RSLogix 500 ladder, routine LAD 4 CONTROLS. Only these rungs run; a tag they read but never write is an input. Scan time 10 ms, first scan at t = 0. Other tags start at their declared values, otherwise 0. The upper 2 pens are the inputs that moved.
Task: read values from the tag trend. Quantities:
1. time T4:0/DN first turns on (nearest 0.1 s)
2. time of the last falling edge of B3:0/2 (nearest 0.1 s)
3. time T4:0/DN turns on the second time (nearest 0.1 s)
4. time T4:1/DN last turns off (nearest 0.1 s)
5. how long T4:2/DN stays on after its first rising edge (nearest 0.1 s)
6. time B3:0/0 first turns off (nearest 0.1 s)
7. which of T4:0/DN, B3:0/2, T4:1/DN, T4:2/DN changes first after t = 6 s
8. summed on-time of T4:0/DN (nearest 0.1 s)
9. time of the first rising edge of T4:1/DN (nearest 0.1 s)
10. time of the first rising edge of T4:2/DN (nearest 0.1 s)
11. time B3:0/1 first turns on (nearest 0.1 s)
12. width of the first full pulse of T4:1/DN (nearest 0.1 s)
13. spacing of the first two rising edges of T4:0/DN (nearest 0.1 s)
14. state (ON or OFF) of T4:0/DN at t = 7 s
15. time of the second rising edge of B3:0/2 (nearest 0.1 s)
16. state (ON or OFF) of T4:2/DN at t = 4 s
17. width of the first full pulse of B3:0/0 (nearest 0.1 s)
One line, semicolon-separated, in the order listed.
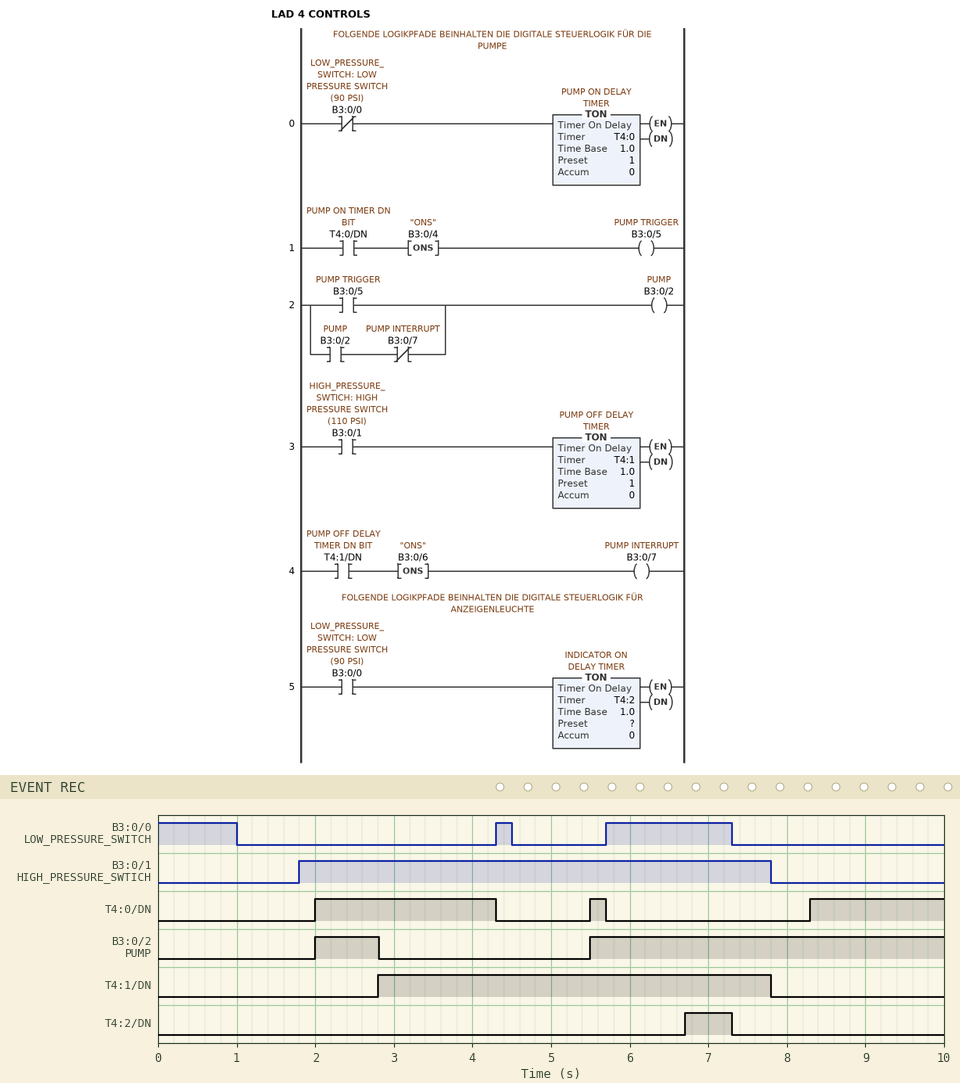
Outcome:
2.0 s; 2.8 s; 5.5 s; 7.8 s; 0.6 s; 1.0 s; T4:2/DN; 4.2 s; 2.8 s; 6.7 s; 1.8 s; 5.0 s; 3.5 s; OFF; 5.5 s; OFF; 0.2 s
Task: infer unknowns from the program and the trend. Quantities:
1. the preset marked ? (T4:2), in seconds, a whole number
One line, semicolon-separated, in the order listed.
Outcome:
1 s
